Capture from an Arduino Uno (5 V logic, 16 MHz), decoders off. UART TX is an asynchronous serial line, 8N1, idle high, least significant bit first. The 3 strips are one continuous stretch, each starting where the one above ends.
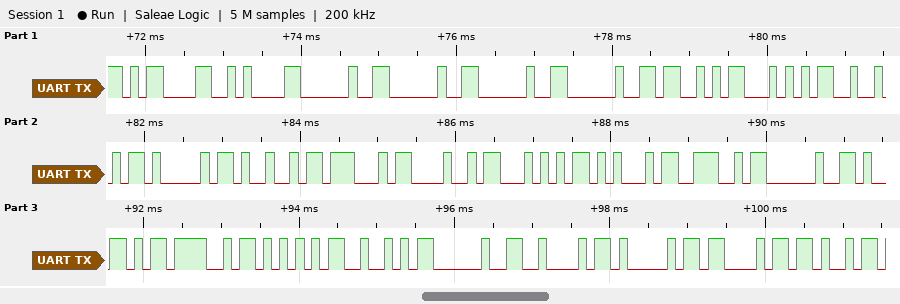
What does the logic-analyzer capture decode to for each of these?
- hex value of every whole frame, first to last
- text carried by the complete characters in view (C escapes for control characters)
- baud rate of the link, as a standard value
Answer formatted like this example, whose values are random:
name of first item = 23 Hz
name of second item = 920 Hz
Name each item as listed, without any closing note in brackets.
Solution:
hex value of every whole frame, first to last = 0D 0A 20 20 20 20 53 54 52 41 49 47 48 54 45 4E 20 59 4F 55 52 20 42 41 43 4B
text carried by the complete characters in view = "\r\n    STRAIGHTEN YOUR BACK"
baud rate of the link, as a standard value = 9600 baud
